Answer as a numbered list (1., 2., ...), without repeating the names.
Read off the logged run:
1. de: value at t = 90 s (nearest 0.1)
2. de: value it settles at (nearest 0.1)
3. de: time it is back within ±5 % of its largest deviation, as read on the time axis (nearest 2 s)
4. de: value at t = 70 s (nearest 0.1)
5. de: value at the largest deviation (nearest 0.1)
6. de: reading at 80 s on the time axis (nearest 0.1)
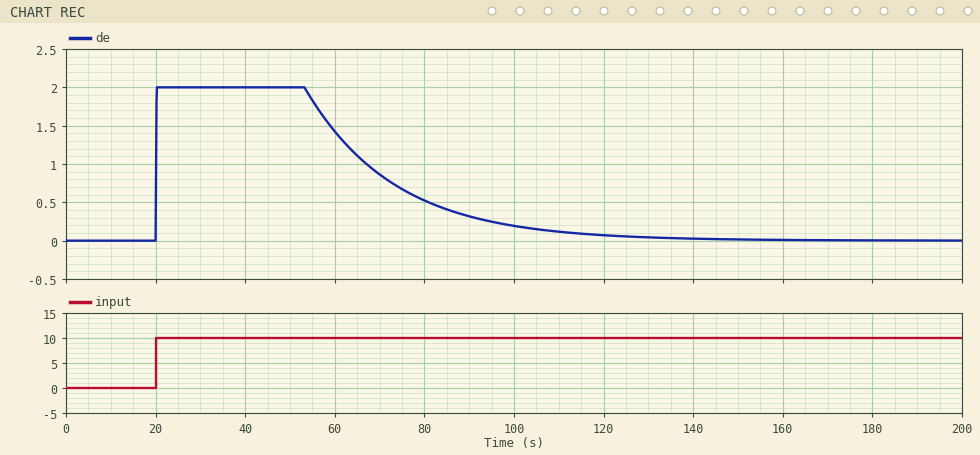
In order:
1. 0.3
2. 0.0
3. 114 s
4. 0.9
5. 2.0
6. 0.5
